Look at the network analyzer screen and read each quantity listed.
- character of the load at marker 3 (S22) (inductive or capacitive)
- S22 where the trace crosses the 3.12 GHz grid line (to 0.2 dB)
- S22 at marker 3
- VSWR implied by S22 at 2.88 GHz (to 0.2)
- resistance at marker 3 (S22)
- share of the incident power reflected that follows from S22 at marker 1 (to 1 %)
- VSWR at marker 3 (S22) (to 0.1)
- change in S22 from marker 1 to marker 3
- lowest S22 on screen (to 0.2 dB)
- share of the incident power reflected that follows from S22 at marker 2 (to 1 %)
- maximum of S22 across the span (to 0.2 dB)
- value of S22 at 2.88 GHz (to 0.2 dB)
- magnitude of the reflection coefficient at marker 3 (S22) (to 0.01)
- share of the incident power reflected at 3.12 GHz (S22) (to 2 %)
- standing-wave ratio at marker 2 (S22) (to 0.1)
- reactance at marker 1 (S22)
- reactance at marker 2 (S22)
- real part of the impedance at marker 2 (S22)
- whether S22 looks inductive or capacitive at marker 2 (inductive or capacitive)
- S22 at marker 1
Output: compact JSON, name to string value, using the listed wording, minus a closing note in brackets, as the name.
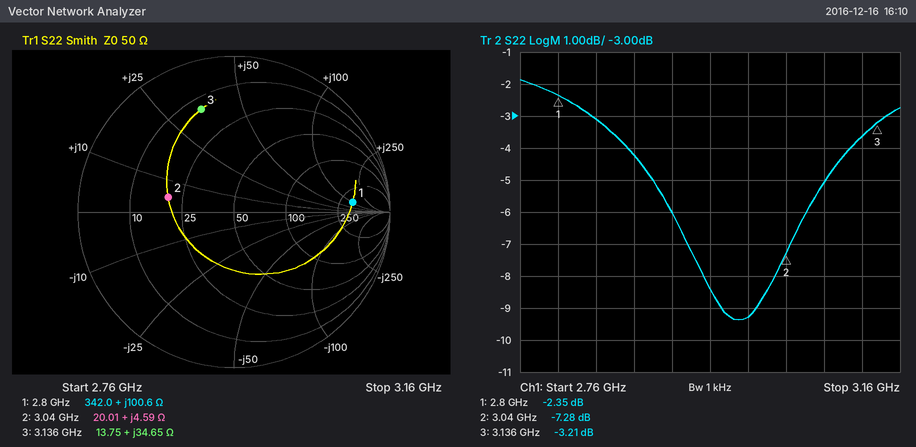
{"character of the load at marker 3 (S22)": "inductive", "S22 where the trace crosses the 3.12 GHz grid line": "-3.6 dB", "S22 at marker 3": "-3.21 dB", "VSWR implied by S22 at 2.88 GHz": "4.2", "resistance at marker 3": "13.75 Ω", "share of the incident power reflected that follows from S22 at marker 1": "58 %", "VSWR at marker 3 (S22)": "5.5", "change in S22 from marker 1 to marker 3": "-0.86 dB", "lowest S22 on screen": "-9.4 dB", "share of the incident power reflected that follows from S22 at marker 2": "19 %", "maximum of S22 across the span": "-1.8 dB", "value of S22 at 2.88 GHz": "-4.2 dB", "magnitude of the reflection coefficient at marker 3 (S22)": "0.69", "share of the incident power reflected at 3.12 GHz (S22)": "44 %", "standing-wave ratio at marker 2 (S22)": "2.5", "reactance at marker 1": "+100.6 Ω", "reactance at marker 2": "+4.59 Ω", "real part of the impedance at marker 2": "20.01 Ω", "whether S22 looks inductive or capacitive at marker 2": "inductive", "S22 at marker 1": "-2.35 dB"}
